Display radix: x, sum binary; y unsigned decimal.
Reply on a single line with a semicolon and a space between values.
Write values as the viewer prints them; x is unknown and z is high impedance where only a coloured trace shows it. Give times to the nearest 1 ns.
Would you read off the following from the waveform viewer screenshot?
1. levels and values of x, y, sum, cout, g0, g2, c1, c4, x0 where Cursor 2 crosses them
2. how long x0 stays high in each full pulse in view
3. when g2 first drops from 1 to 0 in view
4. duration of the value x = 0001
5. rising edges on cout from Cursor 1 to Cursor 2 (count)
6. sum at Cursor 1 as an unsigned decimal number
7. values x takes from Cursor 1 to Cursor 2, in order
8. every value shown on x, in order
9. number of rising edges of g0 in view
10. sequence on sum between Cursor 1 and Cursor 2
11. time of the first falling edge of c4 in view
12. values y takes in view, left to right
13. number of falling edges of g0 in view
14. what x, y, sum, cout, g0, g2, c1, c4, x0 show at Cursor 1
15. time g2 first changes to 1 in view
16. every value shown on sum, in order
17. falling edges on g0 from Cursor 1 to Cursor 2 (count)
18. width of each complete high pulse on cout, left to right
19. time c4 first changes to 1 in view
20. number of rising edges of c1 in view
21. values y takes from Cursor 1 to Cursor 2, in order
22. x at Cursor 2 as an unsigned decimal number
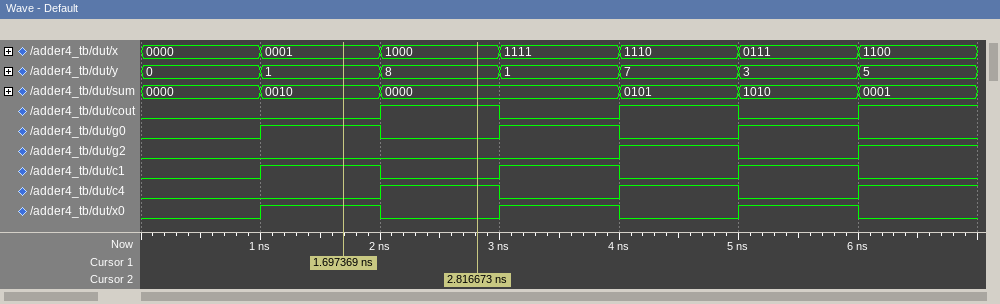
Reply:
x=1000, y=8, sum=0000, cout=1, g0=0, g2=0, c1=0, c4=1, x0=0; 1 ns, 1 ns, 1 ns; 5 ns; 1 ns; 1; 2; 0001, 1000; 0000, 0001, 1000, 1111, 1110, 0111, 1100; 3; 0010, 0000; 3 ns; 0, 1, 8, 1, 7, 3, 5; 3; x=0001, y=1, sum=0010, cout=0, g0=1, g2=0, c1=1, c4=0, x0=1; 4 ns; 0000, 0010, 0000, 0101, 1010, 0001; 1; 1 ns, 1 ns; 2 ns; 3; 1, 8; 8
